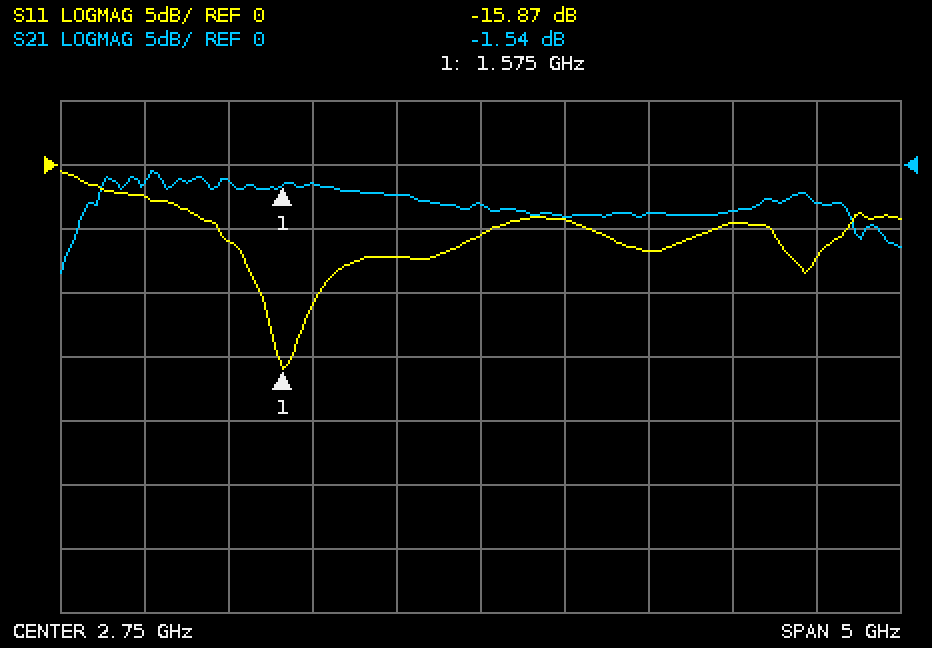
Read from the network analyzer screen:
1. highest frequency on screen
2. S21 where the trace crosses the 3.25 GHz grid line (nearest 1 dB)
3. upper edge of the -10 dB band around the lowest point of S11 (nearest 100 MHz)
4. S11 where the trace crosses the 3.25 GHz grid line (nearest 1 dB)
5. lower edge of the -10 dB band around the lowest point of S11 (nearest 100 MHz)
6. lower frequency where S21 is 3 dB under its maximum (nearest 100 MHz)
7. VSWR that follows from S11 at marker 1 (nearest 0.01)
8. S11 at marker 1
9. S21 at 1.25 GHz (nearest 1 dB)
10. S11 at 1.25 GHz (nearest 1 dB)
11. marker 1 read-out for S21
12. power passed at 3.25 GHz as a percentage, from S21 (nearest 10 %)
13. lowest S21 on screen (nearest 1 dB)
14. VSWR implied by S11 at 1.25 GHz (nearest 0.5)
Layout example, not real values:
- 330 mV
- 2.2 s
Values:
- 5.25 GHz
- -4 dB
- 1.8 GHz
- -4 dB
- 1.4 GHz
- 400 MHz
- 1.38
- -15.87 dB
- -1 dB
- -6 dB
- -1.54 dB
- 40 %
- -8 dB
- 3.0
